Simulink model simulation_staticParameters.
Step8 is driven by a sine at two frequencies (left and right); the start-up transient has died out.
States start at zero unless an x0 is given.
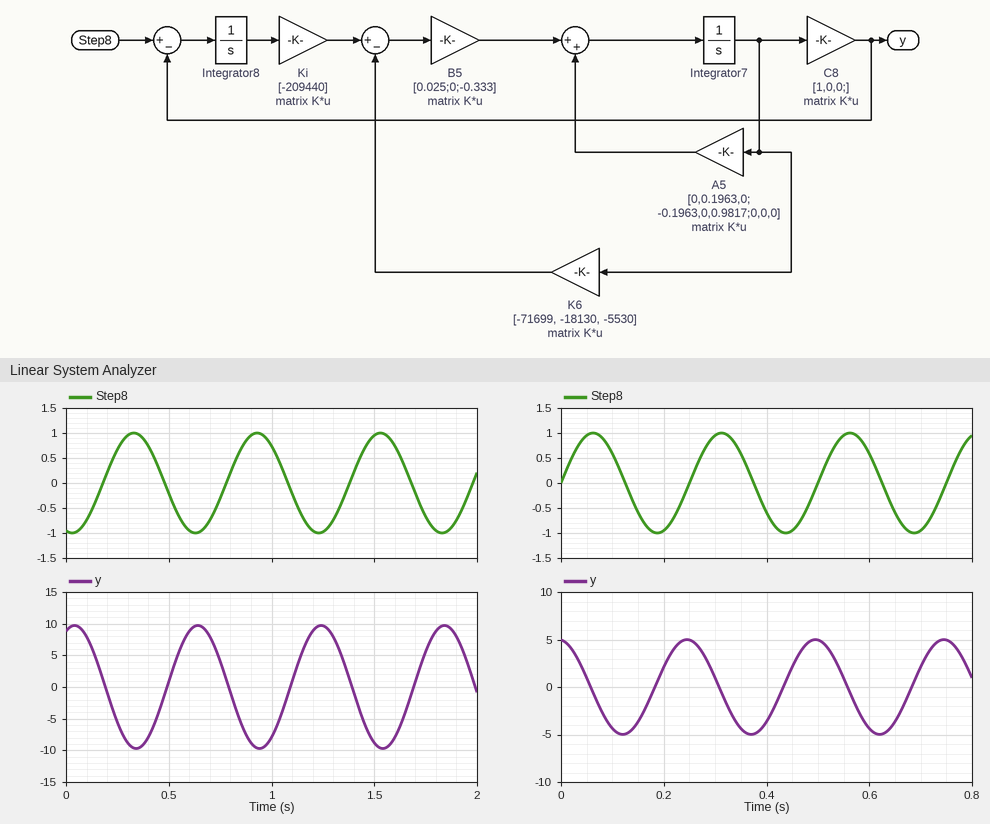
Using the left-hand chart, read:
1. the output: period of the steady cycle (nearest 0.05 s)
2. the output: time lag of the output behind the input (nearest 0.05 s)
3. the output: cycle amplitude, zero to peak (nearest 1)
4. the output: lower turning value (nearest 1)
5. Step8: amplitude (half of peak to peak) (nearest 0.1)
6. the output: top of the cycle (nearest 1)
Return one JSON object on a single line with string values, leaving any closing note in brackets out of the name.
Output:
{"the output: period of the steady cycle": "0.60 s", "the output: time lag of the output behind the input": "0.30 s", "the output: cycle amplitude, zero to peak": "10", "the output: lower turning value": "-10", "Step8: amplitude (half of peak to peak)": "1.0", "the output: top of the cycle": "10"}
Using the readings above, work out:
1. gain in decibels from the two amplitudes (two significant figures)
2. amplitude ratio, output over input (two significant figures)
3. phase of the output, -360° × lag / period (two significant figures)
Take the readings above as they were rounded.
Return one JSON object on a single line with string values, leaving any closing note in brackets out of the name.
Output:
{"gain in decibels from the two amplitudes": "20 dB", "amplitude ratio, output over input": "10", "phase of the output, -360° × lag / period": "-180°"}
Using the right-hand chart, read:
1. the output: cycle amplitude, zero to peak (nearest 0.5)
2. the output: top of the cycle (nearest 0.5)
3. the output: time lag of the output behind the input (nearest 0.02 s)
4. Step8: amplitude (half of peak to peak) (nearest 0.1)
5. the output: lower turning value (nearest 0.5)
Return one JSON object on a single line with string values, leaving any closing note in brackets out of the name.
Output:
{"the output: cycle amplitude, zero to peak": "5.0", "the output: top of the cycle": "5.0", "the output: time lag of the output behind the input": "0.18 s", "Step8: amplitude (half of peak to peak)": "1.0", "the output: lower turning value": "-5.0"}
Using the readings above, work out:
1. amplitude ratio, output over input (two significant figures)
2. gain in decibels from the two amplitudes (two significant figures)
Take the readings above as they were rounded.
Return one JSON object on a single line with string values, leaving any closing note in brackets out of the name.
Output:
{"amplitude ratio, output over input": "5.0", "gain in decibels from the two amplitudes": "14 dB"}
